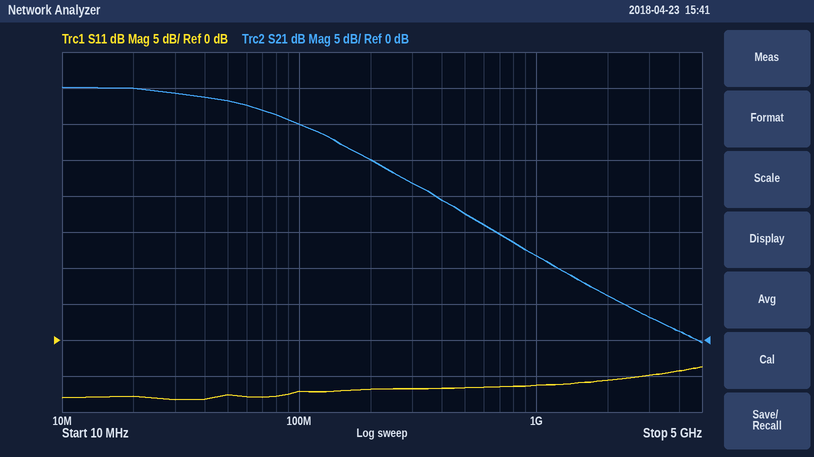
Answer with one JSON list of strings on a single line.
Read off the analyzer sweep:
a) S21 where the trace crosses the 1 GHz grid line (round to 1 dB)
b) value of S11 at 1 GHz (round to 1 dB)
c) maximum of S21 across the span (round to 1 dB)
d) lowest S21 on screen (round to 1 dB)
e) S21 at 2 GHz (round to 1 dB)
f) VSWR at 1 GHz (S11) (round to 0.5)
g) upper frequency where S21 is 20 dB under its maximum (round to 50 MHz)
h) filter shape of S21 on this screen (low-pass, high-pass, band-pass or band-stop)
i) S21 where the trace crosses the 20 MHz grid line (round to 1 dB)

["12 dB", "-6 dB", "35 dB", "0 dB", "6 dB", "3.0", "650 MHz", "low-pass", "35 dB"]
